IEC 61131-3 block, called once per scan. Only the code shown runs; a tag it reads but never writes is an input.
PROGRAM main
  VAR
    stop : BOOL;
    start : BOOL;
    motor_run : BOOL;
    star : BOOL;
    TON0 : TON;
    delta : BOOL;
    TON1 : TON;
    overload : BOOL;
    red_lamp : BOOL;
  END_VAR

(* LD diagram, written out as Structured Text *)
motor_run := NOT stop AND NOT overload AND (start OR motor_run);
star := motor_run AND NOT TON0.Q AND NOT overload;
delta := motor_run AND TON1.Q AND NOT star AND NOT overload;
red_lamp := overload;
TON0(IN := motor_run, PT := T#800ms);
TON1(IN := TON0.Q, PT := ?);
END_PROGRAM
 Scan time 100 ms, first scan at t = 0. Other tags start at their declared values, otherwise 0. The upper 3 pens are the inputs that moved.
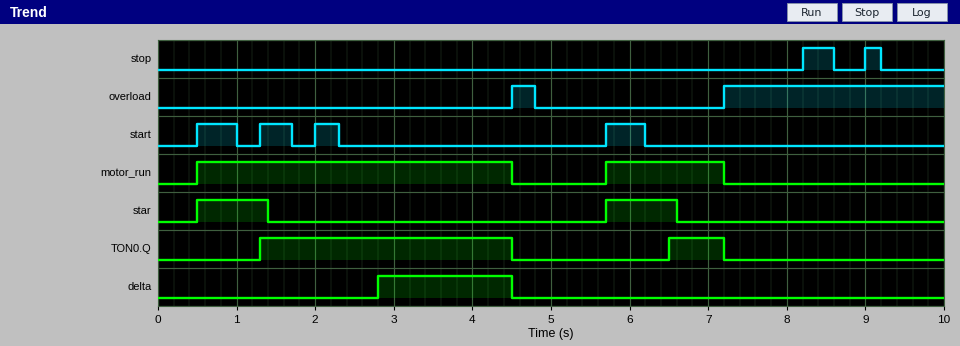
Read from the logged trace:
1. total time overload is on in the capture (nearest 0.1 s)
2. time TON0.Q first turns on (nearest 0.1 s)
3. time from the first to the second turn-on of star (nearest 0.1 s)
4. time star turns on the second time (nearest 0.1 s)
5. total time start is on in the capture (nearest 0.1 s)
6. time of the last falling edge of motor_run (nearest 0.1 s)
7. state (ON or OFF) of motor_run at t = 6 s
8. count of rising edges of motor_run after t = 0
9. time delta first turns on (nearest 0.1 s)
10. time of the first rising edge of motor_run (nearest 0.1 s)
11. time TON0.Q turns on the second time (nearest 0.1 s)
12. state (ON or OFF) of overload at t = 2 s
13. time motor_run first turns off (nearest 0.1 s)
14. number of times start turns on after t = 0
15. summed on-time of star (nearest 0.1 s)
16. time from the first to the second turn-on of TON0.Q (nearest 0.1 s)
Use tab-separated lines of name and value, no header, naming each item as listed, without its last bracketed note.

total time overload is on in the capture	3.1 s
time TON0.Q first turns on	1.3 s
time from the first to the second turn-on of star	5.2 s
time star turns on the second time	5.7 s
total time start is on in the capture	1.7 s
time of the last falling edge of motor_run	7.2 s
state (ON or OFF) of motor_run at t = 6 s	ON
count of rising edges of motor_run after t = 0	2
time delta first turns on	2.8 s
time of the first rising edge of motor_run	0.5 s
time TON0.Q turns on the second time	6.5 s
state (ON or OFF) of overload at t = 2 s	OFF
time motor_run first turns off	4.5 s
number of times start turns on after t = 0	4
summed on-time of star	1.8 s
time from the first to the second turn-on of TON0.Q	5.2 s
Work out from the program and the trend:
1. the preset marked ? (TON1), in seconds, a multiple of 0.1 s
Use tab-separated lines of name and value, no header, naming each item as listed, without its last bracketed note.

the preset marked ? (TON1), in seconds, a multiple of 0.1 s	1.4 s
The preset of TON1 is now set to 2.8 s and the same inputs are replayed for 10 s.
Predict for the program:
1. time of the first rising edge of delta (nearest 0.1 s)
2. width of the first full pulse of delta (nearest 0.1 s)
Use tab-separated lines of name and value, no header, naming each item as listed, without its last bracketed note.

time of the first rising edge of delta	4.2 s
width of the first full pulse of delta	0.3 s
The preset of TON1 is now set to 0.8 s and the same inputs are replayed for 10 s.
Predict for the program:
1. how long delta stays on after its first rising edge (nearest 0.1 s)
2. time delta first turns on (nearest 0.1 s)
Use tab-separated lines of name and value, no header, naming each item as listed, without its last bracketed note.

how long delta stays on after its first rising edge	2.3 s
time delta first turns on	2.2 s
